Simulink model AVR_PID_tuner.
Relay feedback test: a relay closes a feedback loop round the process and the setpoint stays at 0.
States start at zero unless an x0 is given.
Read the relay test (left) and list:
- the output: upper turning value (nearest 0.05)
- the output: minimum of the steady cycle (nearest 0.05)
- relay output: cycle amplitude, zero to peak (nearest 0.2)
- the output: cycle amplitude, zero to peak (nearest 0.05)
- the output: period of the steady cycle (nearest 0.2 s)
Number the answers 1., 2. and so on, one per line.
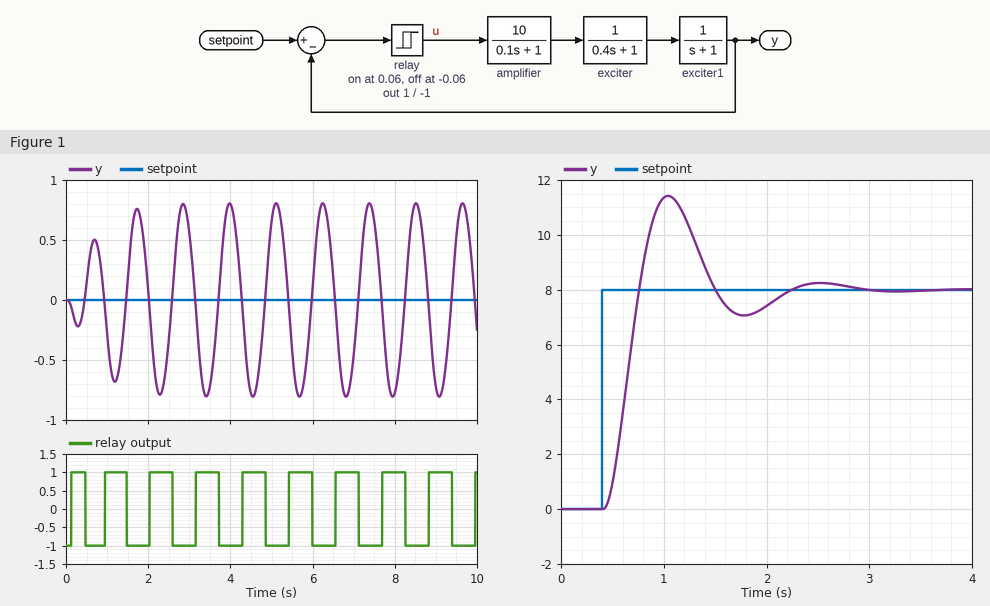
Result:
1. 0.80
2. -0.80
3. 1.0
4. 0.80
5. 1.2 s
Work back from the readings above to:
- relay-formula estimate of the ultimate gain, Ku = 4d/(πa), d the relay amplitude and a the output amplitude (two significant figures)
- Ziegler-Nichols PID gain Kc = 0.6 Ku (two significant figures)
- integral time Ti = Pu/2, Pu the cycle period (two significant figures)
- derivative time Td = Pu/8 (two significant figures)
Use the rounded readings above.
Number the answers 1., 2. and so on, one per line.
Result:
1. 1.6
2. 0.96
3. 0.60 s
4. 0.15 s
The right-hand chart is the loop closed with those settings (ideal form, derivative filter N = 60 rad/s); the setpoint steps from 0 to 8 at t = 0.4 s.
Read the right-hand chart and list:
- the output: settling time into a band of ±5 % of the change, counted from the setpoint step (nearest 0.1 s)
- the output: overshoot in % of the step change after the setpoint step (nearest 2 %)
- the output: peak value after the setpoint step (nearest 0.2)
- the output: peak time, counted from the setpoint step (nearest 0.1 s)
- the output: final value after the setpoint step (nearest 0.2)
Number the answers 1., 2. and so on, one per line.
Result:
1. 1.7 s
2. 42 %
3. 11.4
4. 0.6 s
5. 8.0
